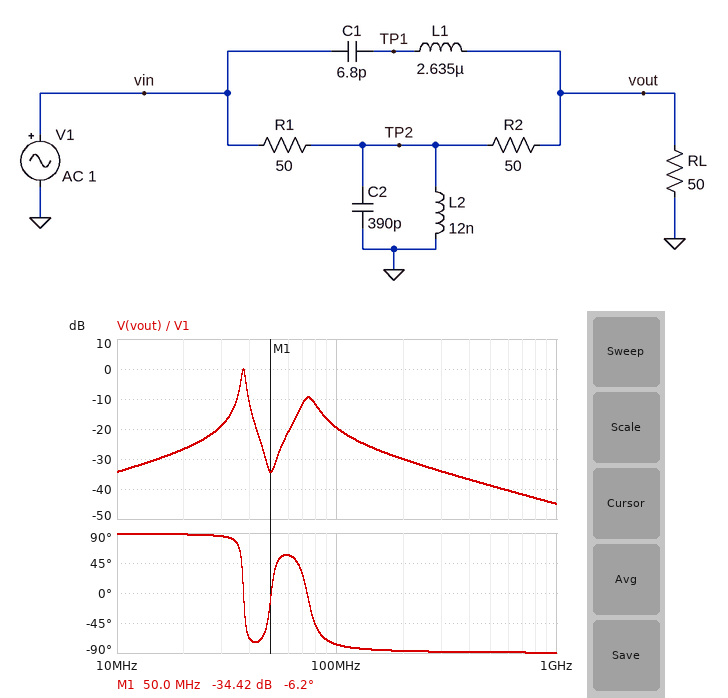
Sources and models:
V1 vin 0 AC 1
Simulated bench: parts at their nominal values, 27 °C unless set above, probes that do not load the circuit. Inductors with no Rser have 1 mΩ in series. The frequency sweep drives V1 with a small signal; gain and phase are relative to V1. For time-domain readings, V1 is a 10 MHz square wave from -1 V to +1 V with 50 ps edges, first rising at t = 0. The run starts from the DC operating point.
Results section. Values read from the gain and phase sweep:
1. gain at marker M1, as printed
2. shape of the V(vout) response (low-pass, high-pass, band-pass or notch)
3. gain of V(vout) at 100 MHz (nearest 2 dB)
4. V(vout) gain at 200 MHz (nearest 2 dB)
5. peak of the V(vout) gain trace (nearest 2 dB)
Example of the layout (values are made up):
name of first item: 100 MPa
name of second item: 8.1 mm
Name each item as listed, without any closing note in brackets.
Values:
gain at marker M1, as printed: -34.42 dB
shape of the V(vout) response: band-pass
gain of V(vout) at 100 MHz: -20 dB
V(vout) gain at 200 MHz: -30 dB
peak of the V(vout) gain trace: 0 dB
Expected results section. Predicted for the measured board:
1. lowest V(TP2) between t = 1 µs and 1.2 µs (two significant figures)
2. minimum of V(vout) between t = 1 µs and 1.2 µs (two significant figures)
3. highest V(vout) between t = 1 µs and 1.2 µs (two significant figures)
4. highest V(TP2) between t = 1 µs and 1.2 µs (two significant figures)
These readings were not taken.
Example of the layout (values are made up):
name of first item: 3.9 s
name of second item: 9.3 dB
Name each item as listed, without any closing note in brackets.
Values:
lowest V(TP2) between t = 1 µs and 1.2 µs: -210 mV
minimum of V(vout) between t = 1 µs and 1.2 µs: -150 mV
highest V(vout) between t = 1 µs and 1.2 µs: 150 mV
highest V(TP2) between t = 1 µs and 1.2 µs: 210 mV
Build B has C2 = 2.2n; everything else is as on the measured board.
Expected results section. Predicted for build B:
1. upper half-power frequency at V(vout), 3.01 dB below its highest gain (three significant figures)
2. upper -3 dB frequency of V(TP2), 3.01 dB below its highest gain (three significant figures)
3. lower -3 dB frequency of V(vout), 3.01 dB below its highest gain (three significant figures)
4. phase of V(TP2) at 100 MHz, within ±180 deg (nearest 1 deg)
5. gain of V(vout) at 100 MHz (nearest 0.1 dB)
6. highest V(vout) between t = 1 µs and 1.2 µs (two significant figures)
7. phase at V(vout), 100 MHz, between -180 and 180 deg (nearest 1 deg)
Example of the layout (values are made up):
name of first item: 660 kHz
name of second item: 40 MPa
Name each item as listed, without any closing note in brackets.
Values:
upper half-power frequency at V(vout), 3.01 dB below its highest gain: 38.5 MHz
upper -3 dB frequency of V(TP2), 3.01 dB below its highest gain: 32.1 MHz
lower -3 dB frequency of V(vout), 3.01 dB below its highest gain: 37.0 MHz
phase of V(TP2) at 100 MHz, within ±180 deg: -90 deg
gain of V(vout) at 100 MHz: -31.8 dB
highest V(vout) between t = 1 µs and 1.2 µs: 170 mV
phase at V(vout), 100 MHz, between -180 and 180 deg: -89 deg
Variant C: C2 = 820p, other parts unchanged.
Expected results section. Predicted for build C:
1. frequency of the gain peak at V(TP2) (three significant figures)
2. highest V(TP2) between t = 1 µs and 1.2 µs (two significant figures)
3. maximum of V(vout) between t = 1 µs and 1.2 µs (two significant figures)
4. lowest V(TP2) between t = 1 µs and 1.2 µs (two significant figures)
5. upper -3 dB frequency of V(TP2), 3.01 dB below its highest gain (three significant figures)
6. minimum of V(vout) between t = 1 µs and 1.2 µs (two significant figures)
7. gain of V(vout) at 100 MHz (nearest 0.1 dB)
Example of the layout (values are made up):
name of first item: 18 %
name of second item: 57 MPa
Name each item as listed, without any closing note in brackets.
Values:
frequency of the gain peak at V(TP2): 50.8 MHz
highest V(TP2) between t = 1 µs and 1.2 µs: 230 mV
maximum of V(vout) between t = 1 µs and 1.2 µs: 160 mV
lowest V(TP2) between t = 1 µs and 1.2 µs: -230 mV
upper -3 dB frequency of V(TP2), 3.01 dB below its highest gain: 53.8 MHz
minimum of V(vout) between t = 1 µs and 1.2 µs: -160 mV
gain of V(vout) at 100 MHz: -27.2 dB
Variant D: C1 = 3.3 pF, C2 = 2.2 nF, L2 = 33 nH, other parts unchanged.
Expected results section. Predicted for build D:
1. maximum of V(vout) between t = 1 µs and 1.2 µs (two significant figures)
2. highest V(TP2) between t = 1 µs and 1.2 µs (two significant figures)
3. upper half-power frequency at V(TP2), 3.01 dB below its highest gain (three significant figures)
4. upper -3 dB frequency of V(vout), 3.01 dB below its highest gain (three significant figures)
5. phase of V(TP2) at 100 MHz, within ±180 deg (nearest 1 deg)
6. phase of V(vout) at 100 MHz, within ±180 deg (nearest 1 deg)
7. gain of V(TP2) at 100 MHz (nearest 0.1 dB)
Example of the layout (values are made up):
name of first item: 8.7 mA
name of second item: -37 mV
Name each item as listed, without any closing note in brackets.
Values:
maximum of V(vout) between t = 1 µs and 1.2 µs: 74 mV
highest V(TP2) between t = 1 µs and 1.2 µs: 86 mV
upper half-power frequency at V(TP2), 3.01 dB below its highest gain: 19.8 MHz
upper -3 dB frequency of V(vout), 3.01 dB below its highest gain: 54.8 MHz
phase of V(TP2) at 100 MHz, within ±180 deg: -90 deg
phase of V(vout) at 100 MHz, within ±180 deg: -89 deg
gain of V(TP2) at 100 MHz: -36.5 dB
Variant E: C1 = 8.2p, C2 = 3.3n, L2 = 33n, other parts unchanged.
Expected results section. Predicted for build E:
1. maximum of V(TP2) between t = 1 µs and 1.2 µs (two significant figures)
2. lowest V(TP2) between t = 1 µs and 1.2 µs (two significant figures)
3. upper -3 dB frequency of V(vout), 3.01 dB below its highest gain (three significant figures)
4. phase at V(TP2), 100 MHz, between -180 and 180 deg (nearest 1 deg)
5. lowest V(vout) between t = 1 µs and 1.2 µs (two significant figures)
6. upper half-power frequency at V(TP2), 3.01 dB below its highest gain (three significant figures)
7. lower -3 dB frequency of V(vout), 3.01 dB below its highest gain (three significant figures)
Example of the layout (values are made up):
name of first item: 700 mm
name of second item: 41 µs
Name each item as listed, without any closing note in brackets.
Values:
maximum of V(TP2) between t = 1 µs and 1.2 µs: 95 mV
lowest V(TP2) between t = 1 µs and 1.2 µs: -94 mV
upper -3 dB frequency of V(vout), 3.01 dB below its highest gain: 35.0 MHz
phase at V(TP2), 100 MHz, between -180 and 180 deg: -90 deg
lowest V(vout) between t = 1 µs and 1.2 µs: -120 mV
upper half-power frequency at V(TP2), 3.01 dB below its highest gain: 16.0 MHz
lower -3 dB frequency of V(vout), 3.01 dB below its highest gain: 33.5 MHz
